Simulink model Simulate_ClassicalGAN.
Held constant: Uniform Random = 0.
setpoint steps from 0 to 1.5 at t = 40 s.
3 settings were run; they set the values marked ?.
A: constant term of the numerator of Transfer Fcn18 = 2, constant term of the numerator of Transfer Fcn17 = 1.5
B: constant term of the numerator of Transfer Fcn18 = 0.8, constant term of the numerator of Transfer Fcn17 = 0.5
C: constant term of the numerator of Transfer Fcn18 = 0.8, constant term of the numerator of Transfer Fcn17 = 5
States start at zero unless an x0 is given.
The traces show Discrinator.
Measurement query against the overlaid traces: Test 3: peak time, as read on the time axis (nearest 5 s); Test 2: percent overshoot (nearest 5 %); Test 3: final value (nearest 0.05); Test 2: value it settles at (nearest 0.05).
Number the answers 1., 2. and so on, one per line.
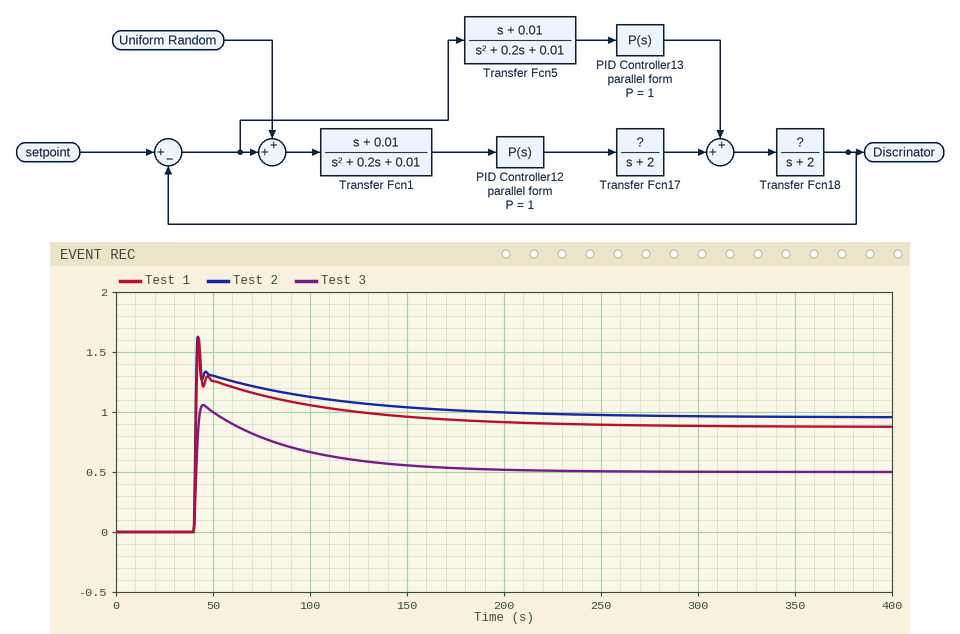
1. 45 s
2. 70 %
3. 0.50
4. 0.95
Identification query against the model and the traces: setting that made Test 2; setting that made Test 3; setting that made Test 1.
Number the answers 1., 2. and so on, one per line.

1. A
2. B
3. C
